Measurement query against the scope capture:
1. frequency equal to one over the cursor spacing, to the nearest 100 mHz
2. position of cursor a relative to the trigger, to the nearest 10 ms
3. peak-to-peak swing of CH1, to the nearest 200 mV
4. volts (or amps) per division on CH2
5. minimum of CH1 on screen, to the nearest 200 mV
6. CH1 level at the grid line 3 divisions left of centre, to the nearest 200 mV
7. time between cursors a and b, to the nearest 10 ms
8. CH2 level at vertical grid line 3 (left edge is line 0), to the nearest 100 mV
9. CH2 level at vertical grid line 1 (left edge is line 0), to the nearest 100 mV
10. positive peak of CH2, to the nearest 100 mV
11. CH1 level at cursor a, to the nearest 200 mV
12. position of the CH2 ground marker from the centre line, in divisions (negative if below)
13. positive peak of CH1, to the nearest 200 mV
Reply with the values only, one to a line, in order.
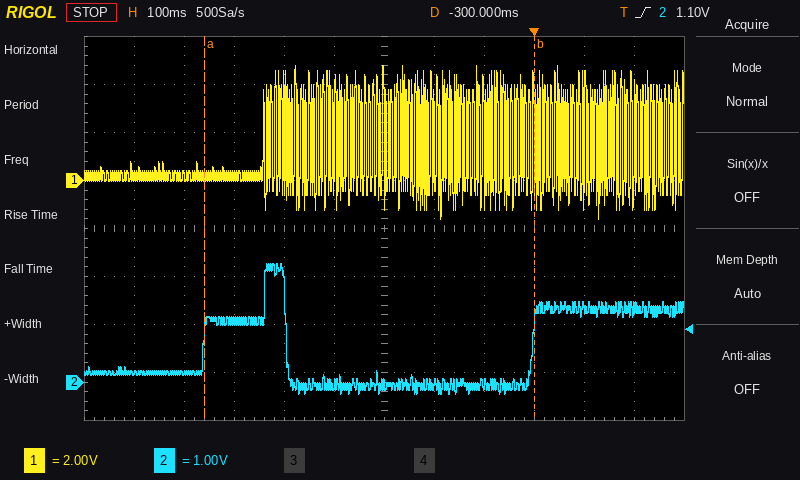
1.5 Hz
-660 ms
6.4 V
1 V
-1.6 V
200 mV
660 ms
1.3 V
200 mV
2.5 V
200 mV
-3.2 div
4.8 V
